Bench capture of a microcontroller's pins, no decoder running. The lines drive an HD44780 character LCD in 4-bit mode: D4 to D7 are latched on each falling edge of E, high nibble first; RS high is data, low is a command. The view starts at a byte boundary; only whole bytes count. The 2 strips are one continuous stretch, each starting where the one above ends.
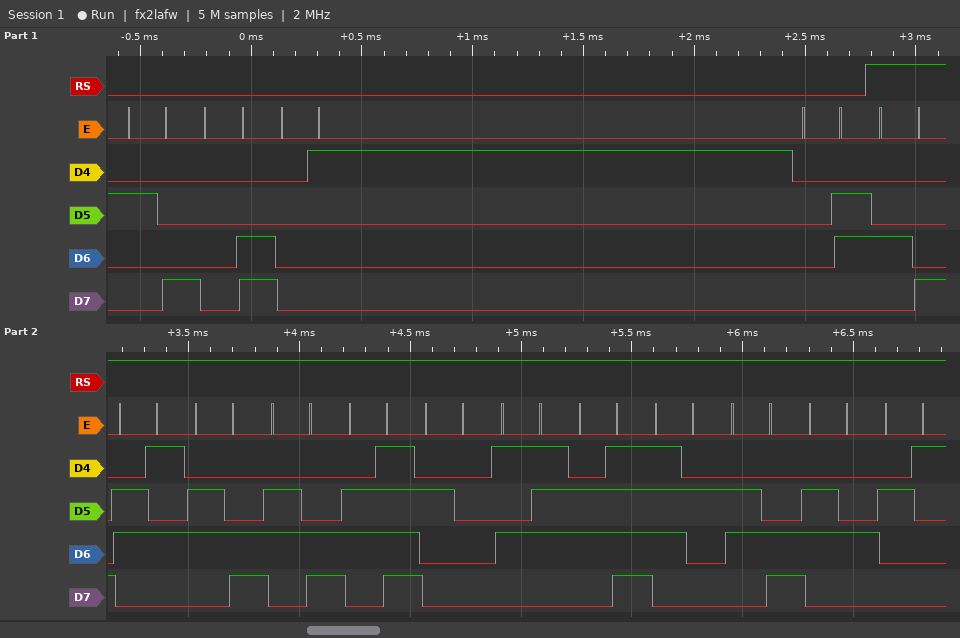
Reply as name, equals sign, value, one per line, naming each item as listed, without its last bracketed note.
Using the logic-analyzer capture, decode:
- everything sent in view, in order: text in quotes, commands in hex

everything sent in view, in order: text in quotes, commands in hex = 0x28 0x0C 0x01 0x06 "Hello World!"
